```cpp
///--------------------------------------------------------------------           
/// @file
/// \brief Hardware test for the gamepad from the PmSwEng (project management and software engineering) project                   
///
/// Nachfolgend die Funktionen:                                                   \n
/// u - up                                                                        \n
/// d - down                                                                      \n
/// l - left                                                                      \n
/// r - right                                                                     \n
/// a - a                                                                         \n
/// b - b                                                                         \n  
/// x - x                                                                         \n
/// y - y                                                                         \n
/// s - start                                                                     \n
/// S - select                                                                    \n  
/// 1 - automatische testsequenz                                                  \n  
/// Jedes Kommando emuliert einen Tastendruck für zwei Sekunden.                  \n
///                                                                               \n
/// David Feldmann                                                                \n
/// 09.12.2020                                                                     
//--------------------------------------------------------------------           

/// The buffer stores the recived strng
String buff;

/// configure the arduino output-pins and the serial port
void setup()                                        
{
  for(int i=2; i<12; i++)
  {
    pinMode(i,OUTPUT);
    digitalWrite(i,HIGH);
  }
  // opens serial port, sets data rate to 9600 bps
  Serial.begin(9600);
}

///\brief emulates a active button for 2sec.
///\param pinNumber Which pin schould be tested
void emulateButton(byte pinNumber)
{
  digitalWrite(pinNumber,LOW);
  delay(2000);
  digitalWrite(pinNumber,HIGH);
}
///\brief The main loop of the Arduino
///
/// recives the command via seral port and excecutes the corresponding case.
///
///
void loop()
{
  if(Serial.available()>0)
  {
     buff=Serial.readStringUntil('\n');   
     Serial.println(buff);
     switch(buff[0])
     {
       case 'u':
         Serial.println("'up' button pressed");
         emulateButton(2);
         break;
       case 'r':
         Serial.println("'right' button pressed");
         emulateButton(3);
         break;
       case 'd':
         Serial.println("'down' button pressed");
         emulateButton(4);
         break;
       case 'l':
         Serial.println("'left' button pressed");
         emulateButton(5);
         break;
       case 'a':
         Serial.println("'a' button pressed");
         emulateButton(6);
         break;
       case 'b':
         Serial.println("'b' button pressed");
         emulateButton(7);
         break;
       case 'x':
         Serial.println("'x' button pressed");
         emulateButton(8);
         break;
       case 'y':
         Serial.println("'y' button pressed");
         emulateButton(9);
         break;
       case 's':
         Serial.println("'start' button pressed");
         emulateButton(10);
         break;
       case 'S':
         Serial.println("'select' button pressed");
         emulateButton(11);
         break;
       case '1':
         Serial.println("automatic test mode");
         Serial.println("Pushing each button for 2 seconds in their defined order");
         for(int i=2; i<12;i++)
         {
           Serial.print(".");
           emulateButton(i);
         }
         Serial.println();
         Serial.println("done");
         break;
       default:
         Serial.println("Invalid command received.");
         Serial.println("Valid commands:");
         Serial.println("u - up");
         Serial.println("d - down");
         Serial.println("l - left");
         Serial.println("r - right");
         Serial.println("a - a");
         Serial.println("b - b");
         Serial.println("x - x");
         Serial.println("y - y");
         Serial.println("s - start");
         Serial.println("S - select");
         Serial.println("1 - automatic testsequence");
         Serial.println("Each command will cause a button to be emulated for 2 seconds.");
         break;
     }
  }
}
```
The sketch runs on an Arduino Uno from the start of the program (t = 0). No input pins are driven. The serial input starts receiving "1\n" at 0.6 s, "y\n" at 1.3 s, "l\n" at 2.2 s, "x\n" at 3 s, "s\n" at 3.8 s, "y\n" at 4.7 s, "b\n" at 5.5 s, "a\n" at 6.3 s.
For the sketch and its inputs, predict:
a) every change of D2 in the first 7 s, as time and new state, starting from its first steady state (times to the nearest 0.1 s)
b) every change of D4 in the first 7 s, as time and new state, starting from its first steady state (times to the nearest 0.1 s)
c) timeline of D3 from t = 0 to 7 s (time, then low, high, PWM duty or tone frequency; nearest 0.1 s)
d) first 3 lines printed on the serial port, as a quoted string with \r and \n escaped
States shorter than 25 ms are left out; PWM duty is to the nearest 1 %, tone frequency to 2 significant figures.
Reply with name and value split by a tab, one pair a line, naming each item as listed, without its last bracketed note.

every change of D2 in the first 7 s, as time and new state, starting from its first steady state	0 s high; 0.6 s low; 2.6 s high
every change of D4 in the first 7 s, as time and new state, starting from its first steady state	0 s high; 4.6 s low; 6.6 s high
timeline of D3 from t = 0 to 7 s	0 s high; 2.6 s low; 4.6 s high
first 3 lines printed on the serial port, as a quoted string with \r and \n escaped	"1\r\nautomatic test mode\r\nPushing each button for 2 seconds in their defined order\r\n"
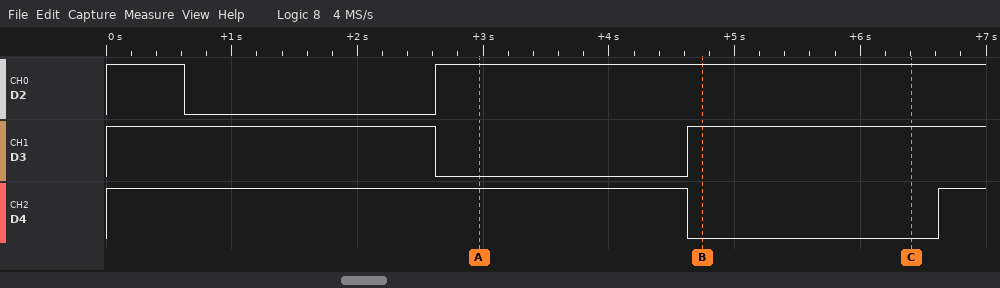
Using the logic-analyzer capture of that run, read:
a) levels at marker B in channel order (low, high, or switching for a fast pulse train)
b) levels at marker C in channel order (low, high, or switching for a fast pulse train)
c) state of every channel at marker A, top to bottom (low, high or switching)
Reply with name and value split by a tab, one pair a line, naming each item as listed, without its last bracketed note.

levels at marker B in channel order	D2 high, D3 high, D4 low
levels at marker C in channel order	D2 high, D3 high, D4 low
state of every channel at marker A, top to bottom	D2 high, D3 low, D4 high
